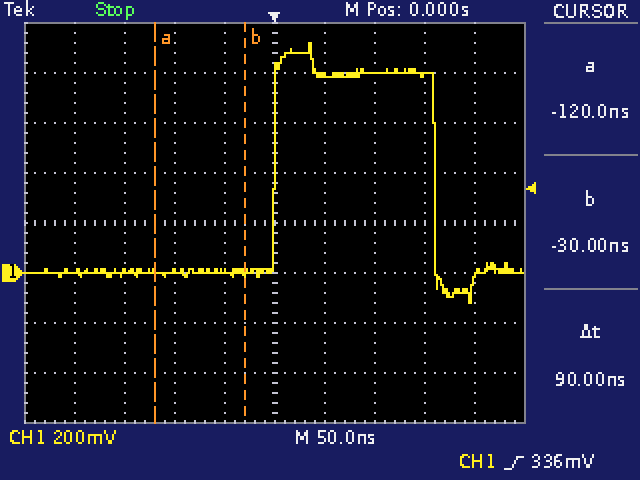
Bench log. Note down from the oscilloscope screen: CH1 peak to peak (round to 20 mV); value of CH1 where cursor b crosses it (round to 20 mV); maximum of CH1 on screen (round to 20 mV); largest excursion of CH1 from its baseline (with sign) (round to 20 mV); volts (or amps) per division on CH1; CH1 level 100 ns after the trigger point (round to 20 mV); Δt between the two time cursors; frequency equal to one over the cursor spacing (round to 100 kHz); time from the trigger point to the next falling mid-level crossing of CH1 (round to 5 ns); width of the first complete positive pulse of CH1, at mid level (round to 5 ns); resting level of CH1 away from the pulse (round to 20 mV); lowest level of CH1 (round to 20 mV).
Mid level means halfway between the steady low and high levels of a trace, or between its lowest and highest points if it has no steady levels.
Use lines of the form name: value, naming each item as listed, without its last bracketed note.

CH1 peak to peak: 1.04 V
value of CH1 where cursor b crosses it: 0 mV
maximum of CH1 on screen: 920 mV
largest excursion of CH1 from its baseline (with sign): +920 mV
volts (or amps) per division on CH1: 200 mV
CH1 level 100 ns after the trigger point: 800 mV
Δt between the two time cursors: 90 ns
frequency equal to one over the cursor spacing: 11.1 MHz
time from the trigger point to the next falling mid-level crossing of CH1: 160 ns
width of the first complete positive pulse of CH1, at mid level: 160 ns
resting level of CH1 away from the pulse: 0 mV
lowest level of CH1: -120 mV
